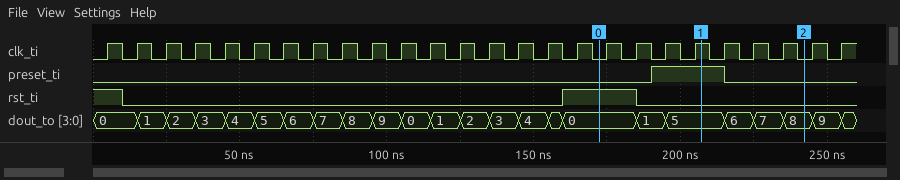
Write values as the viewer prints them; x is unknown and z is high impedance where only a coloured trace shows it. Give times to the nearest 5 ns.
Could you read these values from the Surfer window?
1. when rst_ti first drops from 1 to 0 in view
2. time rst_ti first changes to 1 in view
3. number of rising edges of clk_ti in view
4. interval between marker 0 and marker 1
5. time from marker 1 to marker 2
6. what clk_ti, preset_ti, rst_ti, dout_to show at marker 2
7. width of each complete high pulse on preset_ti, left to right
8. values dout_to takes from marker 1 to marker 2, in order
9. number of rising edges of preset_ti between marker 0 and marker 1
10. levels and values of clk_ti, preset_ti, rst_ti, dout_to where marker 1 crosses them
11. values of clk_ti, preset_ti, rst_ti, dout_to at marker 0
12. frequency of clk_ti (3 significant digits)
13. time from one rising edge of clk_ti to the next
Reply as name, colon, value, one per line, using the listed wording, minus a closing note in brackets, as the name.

when rst_ti first drops from 1 to 0 in view: 10 ns
time rst_ti first changes to 1 in view: 160 ns
number of rising edges of clk_ti in view: 26
interval between marker 0 and marker 1: 35 ns
time from marker 1 to marker 2: 35 ns
what clk_ti, preset_ti, rst_ti, dout_to show at marker 2: clk_ti=0, preset_ti=0, rst_ti=0, dout_to=8
width of each complete high pulse on preset_ti, left to right: 25 ns
values dout_to takes from marker 1 to marker 2, in order: 5, 6, 7, 8
number of rising edges of preset_ti between marker 0 and marker 1: 1
levels and values of clk_ti, preset_ti, rst_ti, dout_to where marker 1 crosses them: clk_ti=1, preset_ti=1, rst_ti=0, dout_to=5
values of clk_ti, preset_ti, rst_ti, dout_to at marker 0: clk_ti=0, preset_ti=0, rst_ti=1, dout_to=0
frequency of clk_ti: 100 MHz
time from one rising edge of clk_ti to the next: 10 ns
